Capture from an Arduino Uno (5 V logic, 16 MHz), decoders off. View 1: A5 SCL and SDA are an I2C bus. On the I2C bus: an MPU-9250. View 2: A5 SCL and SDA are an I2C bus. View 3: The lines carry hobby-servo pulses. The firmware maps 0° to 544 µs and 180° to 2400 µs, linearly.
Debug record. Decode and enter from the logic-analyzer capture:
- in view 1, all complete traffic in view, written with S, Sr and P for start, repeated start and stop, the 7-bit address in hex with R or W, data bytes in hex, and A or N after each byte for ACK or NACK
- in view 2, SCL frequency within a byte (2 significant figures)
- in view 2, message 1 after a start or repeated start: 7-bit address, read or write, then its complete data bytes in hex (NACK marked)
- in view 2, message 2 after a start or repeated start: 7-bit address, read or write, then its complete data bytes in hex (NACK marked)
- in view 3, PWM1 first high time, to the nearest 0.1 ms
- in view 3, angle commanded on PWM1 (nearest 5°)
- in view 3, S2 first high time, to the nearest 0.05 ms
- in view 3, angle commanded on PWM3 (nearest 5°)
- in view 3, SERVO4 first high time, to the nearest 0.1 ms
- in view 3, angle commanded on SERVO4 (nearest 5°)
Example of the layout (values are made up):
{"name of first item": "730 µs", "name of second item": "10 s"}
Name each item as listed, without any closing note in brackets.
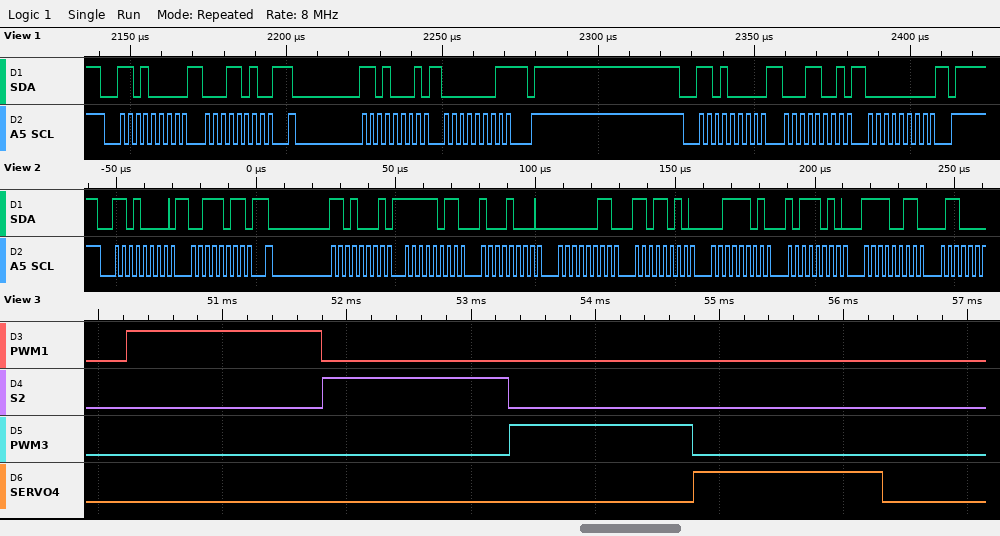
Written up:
{"in view 1, all complete traffic in view, written with S, Sr and P for start, repeated start and stop, the 7-bit address in hex with R or W, data bytes in hex, and A or N after each byte for ACK or NACK": "S 68W A 1A A Sr 68R A 01 N P S 68W A 19 A 00 A P", "in view 2, SCL frequency within a byte": "400 kHz", "in view 2, message 1 after a start or repeated start: 7-bit address, read or write, then its complete data bytes in hex": "0x68 write: 3B", "in view 2, message 2 after a start or repeated start: 7-bit address, read or write, then its complete data bytes in hex": "0x68 read: FB 88 03 DA 3D BA F3", "in view 3, PWM1 first high time, to the nearest 0.1 ms": "1.6 ms", "in view 3, angle commanded on PWM1": "100°", "in view 3, S2 first high time, to the nearest 0.05 ms": "1.50 ms", "in view 3, angle commanded on PWM3": "90°", "in view 3, SERVO4 first high time, to the nearest 0.1 ms": "1.5 ms", "in view 3, angle commanded on SERVO4": "95°"}
